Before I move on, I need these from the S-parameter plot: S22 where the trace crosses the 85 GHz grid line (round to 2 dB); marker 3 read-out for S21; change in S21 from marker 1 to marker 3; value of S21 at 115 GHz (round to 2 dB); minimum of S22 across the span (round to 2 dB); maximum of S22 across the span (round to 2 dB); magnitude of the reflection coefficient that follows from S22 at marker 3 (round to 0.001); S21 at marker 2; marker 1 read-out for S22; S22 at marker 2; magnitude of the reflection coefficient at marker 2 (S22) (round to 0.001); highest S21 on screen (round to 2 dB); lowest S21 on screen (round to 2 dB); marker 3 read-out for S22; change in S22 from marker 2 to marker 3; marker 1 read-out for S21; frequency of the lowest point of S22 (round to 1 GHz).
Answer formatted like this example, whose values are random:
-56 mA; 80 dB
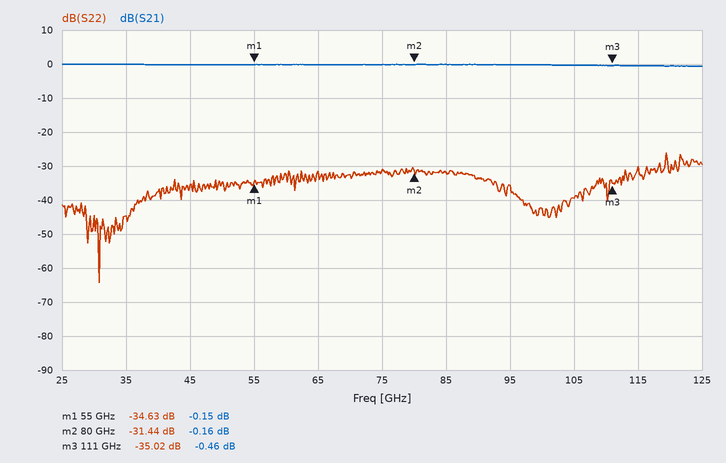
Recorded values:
-32 dB; -0.46 dB; -0.31 dB; 0 dB; -64 dB; -26 dB; 0.018; -0.16 dB; -34.63 dB; -31.44 dB; 0.027; 0 dB; 0 dB; -35.02 dB; -3.58 dB; -0.15 dB; 31 GHz
